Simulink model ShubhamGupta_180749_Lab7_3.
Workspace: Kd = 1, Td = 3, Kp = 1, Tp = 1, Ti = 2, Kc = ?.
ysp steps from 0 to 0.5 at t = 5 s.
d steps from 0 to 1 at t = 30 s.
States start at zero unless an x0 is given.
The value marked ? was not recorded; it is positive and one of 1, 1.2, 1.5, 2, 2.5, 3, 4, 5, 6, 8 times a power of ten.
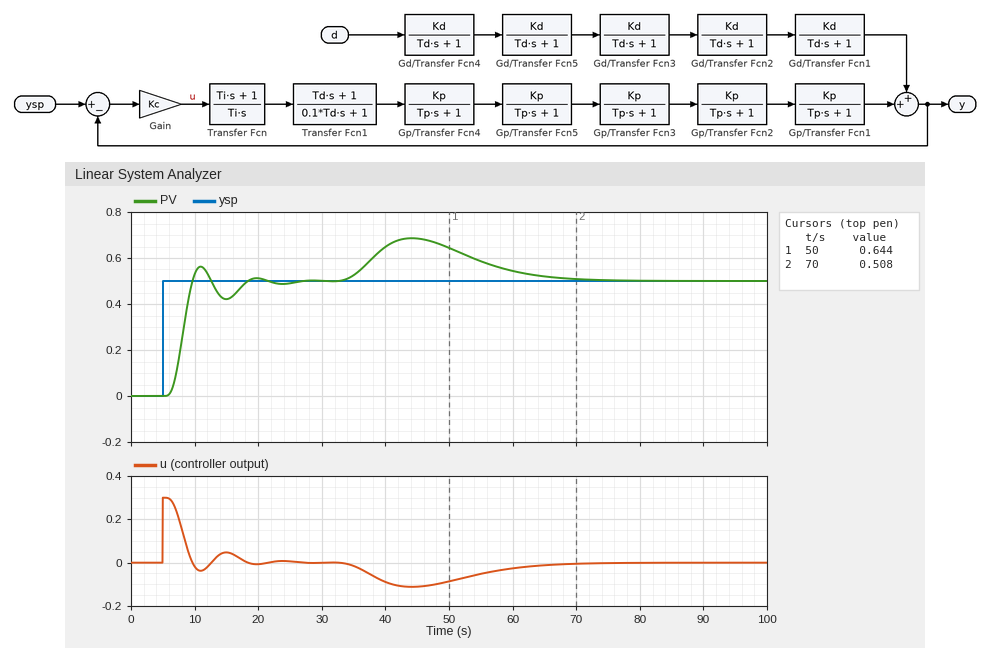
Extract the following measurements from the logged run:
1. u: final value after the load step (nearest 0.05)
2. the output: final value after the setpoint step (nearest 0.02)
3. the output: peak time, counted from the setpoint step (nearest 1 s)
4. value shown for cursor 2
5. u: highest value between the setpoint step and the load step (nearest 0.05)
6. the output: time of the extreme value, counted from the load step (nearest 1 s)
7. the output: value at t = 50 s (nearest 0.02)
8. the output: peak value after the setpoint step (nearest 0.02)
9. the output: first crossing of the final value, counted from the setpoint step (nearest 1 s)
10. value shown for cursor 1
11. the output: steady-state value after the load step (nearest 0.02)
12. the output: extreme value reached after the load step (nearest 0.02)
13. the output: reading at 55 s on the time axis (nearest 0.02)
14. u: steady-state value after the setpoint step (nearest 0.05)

0.00
0.50
6 s
0.508
0.30
14 s
0.64
0.56
5 s
0.644
0.50
0.68
0.58
0.00
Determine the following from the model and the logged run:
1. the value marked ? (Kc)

0.6
